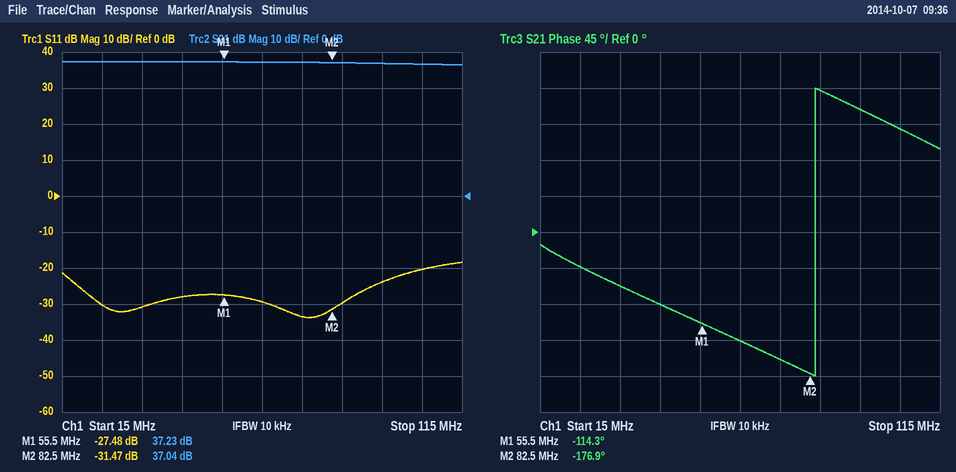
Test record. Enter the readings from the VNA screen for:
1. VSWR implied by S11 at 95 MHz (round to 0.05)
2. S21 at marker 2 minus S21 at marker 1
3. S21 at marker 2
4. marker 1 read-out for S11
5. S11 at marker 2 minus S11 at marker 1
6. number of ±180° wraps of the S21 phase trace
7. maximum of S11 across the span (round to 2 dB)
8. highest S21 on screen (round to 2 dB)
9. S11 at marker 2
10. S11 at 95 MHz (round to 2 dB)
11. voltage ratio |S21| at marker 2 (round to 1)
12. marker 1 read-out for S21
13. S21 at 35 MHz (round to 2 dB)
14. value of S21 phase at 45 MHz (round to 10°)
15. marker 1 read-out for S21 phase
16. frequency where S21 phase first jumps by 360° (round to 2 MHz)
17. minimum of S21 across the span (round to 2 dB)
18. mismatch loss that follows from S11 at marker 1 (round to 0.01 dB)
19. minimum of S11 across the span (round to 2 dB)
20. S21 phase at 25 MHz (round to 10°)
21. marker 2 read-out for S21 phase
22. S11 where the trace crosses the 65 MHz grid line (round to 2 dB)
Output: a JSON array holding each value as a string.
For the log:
["1.15", "-0.19 dB", "37.04 dB", "-27.48 dB", "-3.99 dB", "1", "-18 dB", "38 dB", "-31.47 dB", "-24 dB", "71", "37.23 dB", "38 dB", "-90°", "-114.3°", "84 MHz", "36 dB", "0.01 dB", "-34 dB", "-40°", "-176.9°", "-30 dB"]
